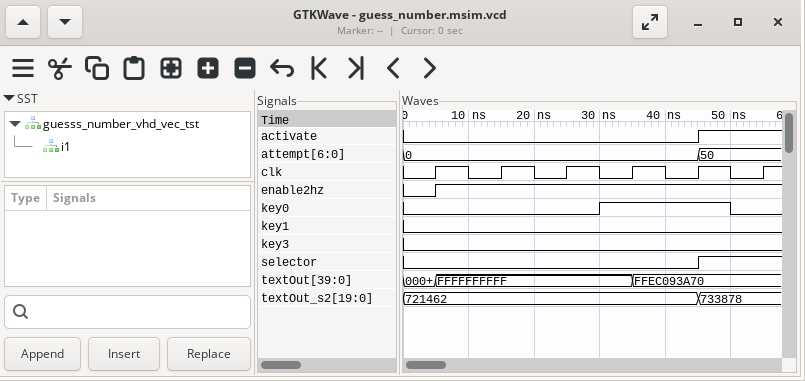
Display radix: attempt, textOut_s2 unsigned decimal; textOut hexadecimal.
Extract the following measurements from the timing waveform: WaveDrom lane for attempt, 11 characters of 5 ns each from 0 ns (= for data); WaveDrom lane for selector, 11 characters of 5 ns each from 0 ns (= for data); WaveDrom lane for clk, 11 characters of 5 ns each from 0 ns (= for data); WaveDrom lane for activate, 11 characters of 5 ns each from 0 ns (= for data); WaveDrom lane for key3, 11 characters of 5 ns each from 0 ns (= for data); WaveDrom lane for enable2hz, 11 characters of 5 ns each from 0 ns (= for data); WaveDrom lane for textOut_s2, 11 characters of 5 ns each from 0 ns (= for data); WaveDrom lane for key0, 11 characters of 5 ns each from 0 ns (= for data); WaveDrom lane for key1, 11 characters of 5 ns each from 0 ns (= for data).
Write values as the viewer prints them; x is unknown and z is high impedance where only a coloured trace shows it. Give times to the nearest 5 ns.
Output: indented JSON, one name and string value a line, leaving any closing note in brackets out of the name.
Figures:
{
  "WaveDrom lane for attempt, 11 characters of 5 ns each from 0 ns": "{name: 'attempt', wave: '=........=.', data: '0 50'}",
  "WaveDrom lane for selector, 11 characters of 5 ns each from 0 ns": "{name: 'selector', wave: '0........1.'}",
  "WaveDrom lane for clk, 11 characters of 5 ns each from 0 ns": "{name: 'clk', wave: '01010101010'}",
  "WaveDrom lane for activate, 11 characters of 5 ns each from 0 ns": "{name: 'activate', wave: '0........1.'}",
  "WaveDrom lane for key3, 11 characters of 5 ns each from 0 ns": "{name: 'key3', wave: '0..........'}",
  "WaveDrom lane for enable2hz, 11 characters of 5 ns each from 0 ns": "{name: 'enable2hz', wave: '01.........'}",
  "WaveDrom lane for textOut_s2, 11 characters of 5 ns each from 0 ns": "{name: 'textOut_s2', wave: '=........=.', data: '721462 733878'}",
  "WaveDrom lane for key0, 11 characters of 5 ns each from 0 ns": "{name: 'key0', wave: '0.....1...0'}",
  "WaveDrom lane for key1, 11 characters of 5 ns each from 0 ns": "{name: 'key1', wave: '0..........'}"
}
